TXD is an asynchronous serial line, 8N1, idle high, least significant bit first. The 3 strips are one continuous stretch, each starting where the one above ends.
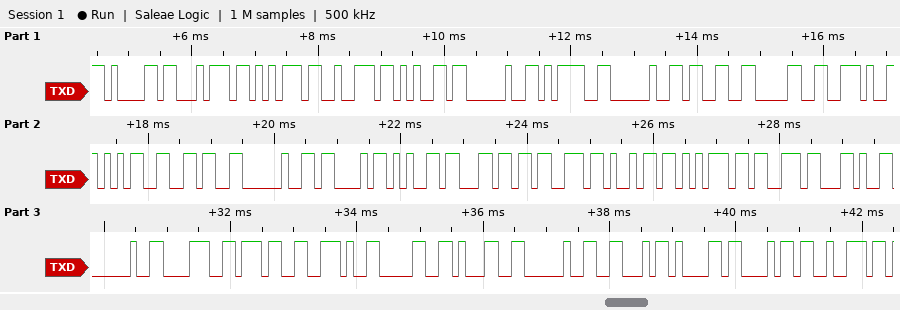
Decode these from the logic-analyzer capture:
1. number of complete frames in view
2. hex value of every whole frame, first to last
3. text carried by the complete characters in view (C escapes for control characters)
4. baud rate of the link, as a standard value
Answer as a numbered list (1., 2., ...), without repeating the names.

1. 33
2. 61 74 75 72 65 20 3D 20 33 30 2E 35 36 20 43 65 6C 73 69 75 73 2C 20 38 37 2E 30 31 20 46 61 68 72
3. "ature = 30.56 Celsius, 87.01 Fahr"
4. 9600 baud
